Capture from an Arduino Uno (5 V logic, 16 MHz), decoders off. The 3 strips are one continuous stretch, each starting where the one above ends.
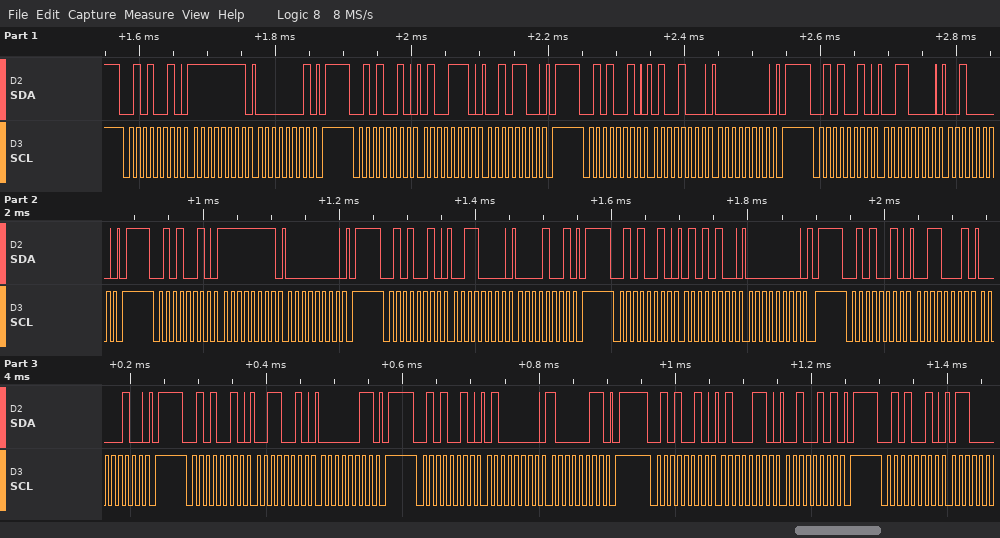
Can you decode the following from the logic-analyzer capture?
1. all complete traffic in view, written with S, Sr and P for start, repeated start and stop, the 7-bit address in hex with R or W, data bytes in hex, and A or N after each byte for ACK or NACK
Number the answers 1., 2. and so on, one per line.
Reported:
1. S 29W A FF A 01 A P S 29W A 4E A 2C A P S 29W A 48 A 00 A P S 29W A 30 A 20 A P S 29W A FF A 00 A P S 29W A 30 A 09 A P S 29W A 54 A 00 A P S 29W A 31 A 04 A P S 29W A 32 A 03 A P S 29W A 40 A 83 A P S 29W A 46 A 25 A P S 29W A
